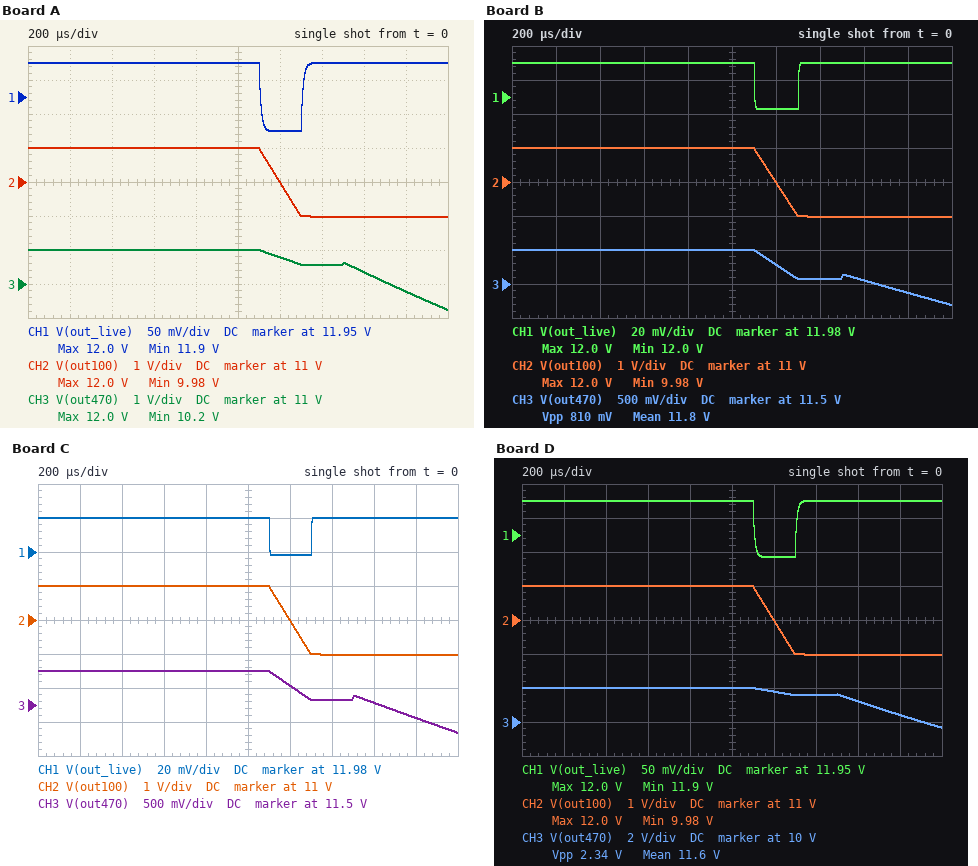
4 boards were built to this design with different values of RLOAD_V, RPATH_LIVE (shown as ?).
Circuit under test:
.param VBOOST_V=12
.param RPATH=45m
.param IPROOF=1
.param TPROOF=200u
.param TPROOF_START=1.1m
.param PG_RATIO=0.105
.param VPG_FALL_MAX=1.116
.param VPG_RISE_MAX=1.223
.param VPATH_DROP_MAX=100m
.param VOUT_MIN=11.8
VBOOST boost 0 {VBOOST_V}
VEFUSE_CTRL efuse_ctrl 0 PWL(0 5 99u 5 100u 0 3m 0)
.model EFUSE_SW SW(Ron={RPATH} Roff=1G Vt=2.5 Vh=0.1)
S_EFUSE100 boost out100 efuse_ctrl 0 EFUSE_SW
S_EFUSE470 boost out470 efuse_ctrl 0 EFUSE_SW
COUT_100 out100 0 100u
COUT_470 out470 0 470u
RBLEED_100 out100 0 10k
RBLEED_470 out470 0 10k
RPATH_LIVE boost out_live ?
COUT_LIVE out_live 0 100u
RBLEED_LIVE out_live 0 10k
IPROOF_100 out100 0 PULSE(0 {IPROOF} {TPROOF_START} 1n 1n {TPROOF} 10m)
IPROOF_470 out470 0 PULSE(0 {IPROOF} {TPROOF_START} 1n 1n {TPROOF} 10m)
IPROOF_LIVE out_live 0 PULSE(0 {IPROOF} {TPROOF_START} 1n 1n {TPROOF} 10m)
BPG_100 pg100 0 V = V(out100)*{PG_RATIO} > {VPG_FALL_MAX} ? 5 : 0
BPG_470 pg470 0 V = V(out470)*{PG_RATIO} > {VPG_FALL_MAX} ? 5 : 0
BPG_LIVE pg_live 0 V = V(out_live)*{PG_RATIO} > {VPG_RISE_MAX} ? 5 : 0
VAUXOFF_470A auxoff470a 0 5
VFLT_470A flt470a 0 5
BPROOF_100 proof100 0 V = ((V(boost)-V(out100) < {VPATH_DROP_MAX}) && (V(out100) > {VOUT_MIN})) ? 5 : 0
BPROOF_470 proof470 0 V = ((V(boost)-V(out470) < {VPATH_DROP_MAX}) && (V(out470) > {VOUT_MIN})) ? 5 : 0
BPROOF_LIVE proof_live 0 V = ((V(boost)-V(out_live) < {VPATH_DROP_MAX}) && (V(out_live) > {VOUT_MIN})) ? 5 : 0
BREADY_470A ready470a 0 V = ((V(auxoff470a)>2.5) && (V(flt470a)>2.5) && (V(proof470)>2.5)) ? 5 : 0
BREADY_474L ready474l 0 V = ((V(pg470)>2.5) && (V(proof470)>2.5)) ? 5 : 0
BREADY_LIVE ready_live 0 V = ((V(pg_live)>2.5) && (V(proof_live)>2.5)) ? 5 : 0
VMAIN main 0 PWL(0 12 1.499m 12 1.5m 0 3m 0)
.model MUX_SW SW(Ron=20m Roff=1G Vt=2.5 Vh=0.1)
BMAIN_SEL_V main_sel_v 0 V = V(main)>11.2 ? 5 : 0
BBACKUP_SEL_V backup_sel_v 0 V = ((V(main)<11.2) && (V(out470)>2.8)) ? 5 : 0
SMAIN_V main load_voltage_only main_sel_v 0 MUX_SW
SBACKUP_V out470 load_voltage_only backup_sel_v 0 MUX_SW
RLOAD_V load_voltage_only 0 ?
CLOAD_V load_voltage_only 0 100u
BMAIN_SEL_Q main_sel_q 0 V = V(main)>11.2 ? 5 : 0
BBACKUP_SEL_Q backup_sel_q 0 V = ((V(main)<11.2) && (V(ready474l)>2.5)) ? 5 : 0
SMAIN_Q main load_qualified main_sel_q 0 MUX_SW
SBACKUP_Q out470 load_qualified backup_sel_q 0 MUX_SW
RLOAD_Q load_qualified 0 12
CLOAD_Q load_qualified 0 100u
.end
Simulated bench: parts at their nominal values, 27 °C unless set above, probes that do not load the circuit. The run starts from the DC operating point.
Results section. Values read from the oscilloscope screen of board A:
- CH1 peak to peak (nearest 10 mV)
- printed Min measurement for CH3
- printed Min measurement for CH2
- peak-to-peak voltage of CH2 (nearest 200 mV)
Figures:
100 mV
10.2 V
9.98 V
2.0 V
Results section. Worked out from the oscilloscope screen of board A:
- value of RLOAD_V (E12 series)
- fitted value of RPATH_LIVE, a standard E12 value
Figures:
6.8 Ω
0.1 Ω
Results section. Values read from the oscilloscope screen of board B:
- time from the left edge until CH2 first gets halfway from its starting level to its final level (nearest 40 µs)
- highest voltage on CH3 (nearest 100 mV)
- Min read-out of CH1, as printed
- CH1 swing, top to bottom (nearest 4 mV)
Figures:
1.20 ms
12.0 V
12.0 V
28 mV
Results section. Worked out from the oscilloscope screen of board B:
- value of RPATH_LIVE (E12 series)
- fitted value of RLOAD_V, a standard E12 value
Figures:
0.027 Ω
22 Ω
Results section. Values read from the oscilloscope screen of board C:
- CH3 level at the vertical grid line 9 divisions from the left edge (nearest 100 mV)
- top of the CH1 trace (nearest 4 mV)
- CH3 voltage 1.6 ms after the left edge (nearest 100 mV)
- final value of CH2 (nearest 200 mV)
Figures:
11.3 V
12.000 V
11.5 V
10.0 V
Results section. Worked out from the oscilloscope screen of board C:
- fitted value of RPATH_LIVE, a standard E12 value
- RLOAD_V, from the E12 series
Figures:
0.022 Ω
18 Ω
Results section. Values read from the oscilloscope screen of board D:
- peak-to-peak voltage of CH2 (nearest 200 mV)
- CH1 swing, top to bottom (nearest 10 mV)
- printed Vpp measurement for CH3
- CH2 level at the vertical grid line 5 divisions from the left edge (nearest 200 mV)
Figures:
2.0 V
80 mV
2.34 V
12.0 V
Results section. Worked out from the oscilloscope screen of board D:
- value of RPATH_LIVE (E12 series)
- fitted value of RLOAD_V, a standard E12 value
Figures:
0.082 Ω
4.7 Ω
